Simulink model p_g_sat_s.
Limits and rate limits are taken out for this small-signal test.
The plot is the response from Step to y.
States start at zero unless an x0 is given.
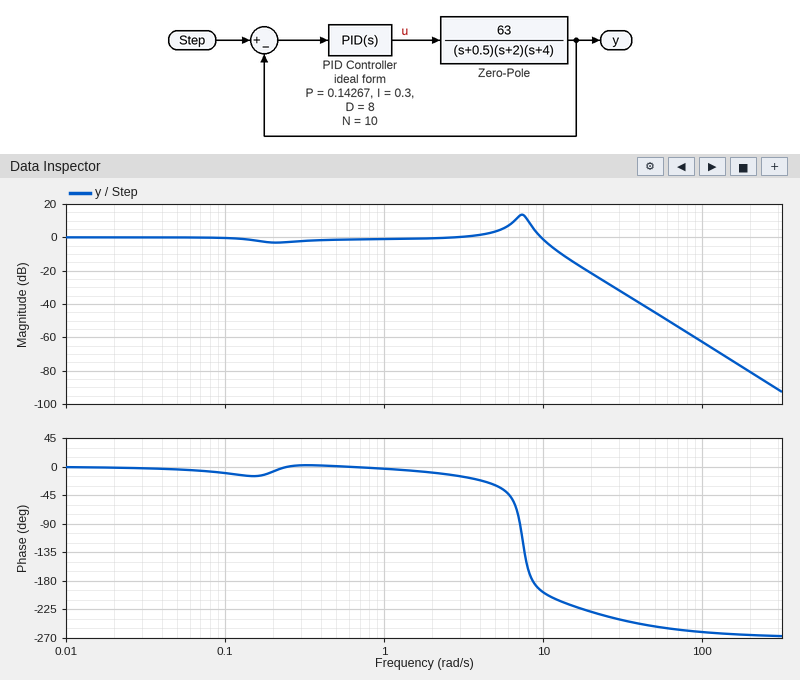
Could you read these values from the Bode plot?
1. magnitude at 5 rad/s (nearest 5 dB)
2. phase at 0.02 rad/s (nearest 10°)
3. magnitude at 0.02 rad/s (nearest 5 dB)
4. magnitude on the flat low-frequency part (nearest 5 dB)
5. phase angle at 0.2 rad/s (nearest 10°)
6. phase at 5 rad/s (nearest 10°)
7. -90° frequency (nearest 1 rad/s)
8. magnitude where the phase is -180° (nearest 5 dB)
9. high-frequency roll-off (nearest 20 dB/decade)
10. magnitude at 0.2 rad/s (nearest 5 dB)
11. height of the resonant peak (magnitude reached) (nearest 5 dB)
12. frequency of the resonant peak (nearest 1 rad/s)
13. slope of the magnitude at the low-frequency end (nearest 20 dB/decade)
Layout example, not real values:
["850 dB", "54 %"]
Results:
["5 dB", "0°", "0 dB", "0 dB", "-10°", "-30°", "7 rad/s", "5 dB", "-60 dB/decade", "-5 dB", "15 dB", "7 rad/s", "0 dB/decade"]
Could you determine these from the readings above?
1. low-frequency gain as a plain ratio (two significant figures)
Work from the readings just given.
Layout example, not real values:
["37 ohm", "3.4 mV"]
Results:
["1.0"]
